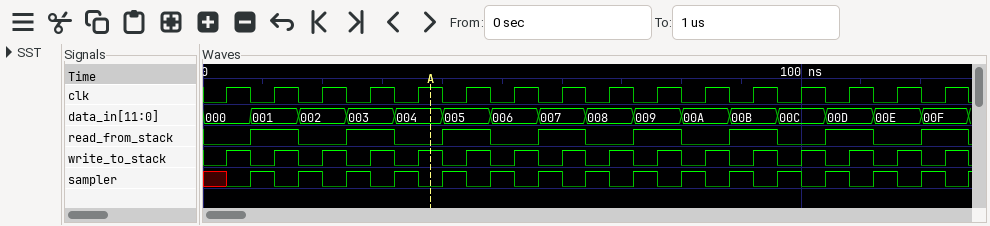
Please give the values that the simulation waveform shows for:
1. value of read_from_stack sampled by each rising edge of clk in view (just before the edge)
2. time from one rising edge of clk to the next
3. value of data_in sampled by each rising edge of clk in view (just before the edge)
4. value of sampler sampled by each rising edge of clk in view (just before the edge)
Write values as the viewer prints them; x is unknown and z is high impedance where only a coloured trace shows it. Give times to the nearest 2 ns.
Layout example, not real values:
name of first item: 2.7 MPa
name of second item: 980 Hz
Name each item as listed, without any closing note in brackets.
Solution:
value of read_from_stack sampled by each rising edge of clk in view: 0 1 0 1 0 1 0 1 0 1 0 1 0 1 0 1
time from one rising edge of clk to the next: 8 ns
value of data_in sampled by each rising edge of clk in view: 000, 001, 002, 003, 004, 005, 006, 007, 008, 009, 00A, 00B, 00C, 00D, 00E, 00F
value of sampler sampled by each rising edge of clk in view: x 1 1 1 1 1 1 1 1 1 1 1 1 1 1 1
